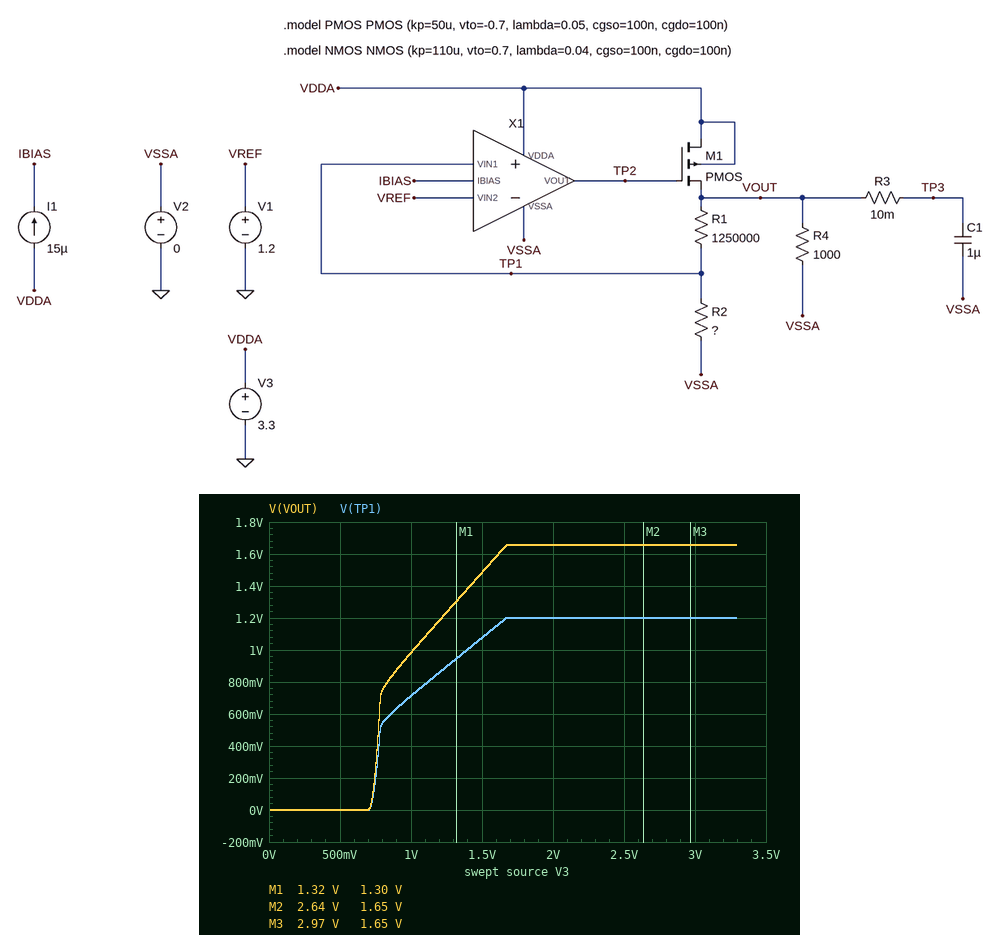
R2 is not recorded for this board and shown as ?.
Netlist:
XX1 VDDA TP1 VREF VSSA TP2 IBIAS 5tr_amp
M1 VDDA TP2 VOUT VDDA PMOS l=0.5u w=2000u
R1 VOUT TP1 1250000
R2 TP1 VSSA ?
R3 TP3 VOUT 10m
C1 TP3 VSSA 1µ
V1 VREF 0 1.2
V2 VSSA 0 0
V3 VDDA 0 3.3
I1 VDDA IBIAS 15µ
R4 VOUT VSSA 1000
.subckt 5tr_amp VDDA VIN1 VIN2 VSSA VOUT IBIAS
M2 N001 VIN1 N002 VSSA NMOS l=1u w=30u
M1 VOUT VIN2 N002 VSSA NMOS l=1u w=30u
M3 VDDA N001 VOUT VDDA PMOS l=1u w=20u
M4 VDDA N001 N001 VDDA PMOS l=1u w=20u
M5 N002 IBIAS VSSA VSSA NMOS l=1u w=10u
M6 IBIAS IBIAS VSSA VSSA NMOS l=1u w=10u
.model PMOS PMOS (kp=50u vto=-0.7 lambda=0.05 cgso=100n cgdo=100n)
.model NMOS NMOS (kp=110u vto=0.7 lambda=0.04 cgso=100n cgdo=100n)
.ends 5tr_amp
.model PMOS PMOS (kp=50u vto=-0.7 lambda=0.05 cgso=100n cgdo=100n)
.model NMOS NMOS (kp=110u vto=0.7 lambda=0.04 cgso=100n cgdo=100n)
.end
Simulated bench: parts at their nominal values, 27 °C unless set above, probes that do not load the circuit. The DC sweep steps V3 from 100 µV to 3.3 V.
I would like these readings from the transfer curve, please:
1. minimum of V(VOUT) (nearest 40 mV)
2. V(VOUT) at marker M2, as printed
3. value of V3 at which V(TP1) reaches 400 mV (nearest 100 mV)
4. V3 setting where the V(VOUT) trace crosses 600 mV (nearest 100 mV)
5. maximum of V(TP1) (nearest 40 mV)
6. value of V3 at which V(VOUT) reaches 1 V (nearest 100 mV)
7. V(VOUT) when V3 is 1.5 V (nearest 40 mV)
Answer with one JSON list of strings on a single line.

["0 V", "1.65 V", "800 mV", "800 mV", "1.20 V", "1.0 V", "1.48 V"]
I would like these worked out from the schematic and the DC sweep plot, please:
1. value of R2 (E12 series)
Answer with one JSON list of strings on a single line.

["3.3 MΩ"]
